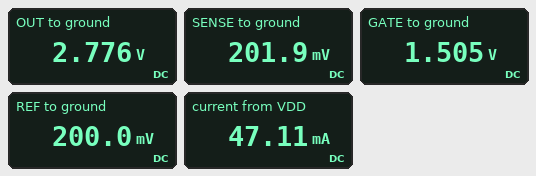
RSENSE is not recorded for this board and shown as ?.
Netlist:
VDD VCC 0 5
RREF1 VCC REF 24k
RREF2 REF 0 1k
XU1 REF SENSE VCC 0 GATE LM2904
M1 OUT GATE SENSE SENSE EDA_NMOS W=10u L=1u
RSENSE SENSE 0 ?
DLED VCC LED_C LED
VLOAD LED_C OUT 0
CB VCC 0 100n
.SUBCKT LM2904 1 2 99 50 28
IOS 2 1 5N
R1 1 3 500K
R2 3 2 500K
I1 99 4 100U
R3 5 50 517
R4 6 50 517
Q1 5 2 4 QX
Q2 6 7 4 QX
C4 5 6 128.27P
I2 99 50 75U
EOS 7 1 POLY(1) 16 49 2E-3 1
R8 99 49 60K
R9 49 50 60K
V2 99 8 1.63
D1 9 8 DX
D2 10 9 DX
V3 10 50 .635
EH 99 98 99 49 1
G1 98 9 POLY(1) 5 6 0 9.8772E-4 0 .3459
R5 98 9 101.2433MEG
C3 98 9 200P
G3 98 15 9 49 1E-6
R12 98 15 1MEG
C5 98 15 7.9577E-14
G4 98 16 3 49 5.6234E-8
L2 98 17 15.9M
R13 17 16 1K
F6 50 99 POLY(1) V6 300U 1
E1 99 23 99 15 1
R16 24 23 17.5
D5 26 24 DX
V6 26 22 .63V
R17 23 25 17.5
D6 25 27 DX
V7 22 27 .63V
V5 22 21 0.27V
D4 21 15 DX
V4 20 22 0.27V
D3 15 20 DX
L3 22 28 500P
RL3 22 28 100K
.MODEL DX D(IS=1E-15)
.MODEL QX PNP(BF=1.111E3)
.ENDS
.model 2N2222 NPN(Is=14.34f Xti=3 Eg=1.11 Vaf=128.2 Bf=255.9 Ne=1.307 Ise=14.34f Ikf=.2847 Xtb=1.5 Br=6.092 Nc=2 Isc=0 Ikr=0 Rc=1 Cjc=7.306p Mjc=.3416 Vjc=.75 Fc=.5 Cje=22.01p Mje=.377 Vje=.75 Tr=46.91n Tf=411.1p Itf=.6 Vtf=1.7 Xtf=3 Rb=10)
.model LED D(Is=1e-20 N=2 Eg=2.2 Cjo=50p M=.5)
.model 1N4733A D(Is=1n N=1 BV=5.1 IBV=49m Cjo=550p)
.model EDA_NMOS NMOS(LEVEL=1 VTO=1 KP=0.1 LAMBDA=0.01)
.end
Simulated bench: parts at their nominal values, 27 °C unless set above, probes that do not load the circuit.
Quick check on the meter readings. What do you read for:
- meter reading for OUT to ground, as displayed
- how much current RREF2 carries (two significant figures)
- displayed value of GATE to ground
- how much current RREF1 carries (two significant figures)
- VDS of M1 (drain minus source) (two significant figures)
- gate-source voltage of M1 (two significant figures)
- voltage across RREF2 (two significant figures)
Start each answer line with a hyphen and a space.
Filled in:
- 2.776 V
- 200 µA
- 1.505 V
- 200 µA
- 2.6 V
- 1.3 V
- 200 mV
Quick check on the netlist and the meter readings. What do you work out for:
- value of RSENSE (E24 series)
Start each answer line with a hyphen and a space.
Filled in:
- 4.3 Ω
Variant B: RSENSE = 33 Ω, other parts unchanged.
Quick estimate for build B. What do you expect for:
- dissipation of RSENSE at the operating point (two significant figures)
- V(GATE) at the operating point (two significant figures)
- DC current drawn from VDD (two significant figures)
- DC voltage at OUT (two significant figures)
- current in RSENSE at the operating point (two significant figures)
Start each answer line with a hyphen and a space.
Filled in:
- 1.2 mW
- 1.3 V
- 6.3 mA
- 2.9 V
- 6.1 mA
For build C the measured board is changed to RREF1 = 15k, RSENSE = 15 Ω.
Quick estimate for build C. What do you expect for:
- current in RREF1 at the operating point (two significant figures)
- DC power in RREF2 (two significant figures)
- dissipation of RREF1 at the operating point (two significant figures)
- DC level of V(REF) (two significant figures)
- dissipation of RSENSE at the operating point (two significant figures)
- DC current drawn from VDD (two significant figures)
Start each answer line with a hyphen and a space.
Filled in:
- 310 µA
- 98 µW
- 1.5 mW
- 310 mV
- 6.6 mW
- 21 mA
